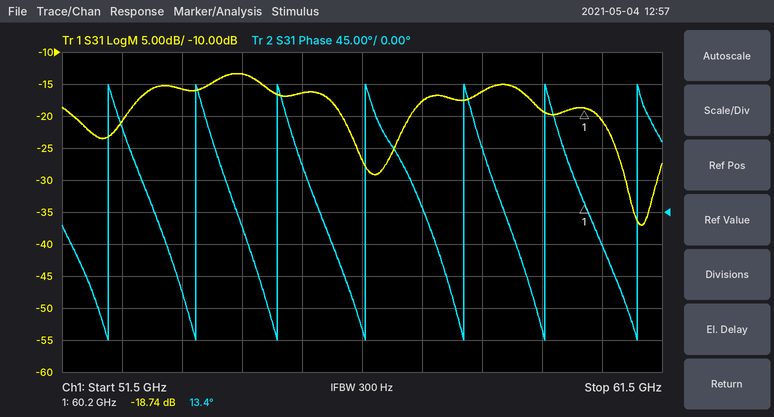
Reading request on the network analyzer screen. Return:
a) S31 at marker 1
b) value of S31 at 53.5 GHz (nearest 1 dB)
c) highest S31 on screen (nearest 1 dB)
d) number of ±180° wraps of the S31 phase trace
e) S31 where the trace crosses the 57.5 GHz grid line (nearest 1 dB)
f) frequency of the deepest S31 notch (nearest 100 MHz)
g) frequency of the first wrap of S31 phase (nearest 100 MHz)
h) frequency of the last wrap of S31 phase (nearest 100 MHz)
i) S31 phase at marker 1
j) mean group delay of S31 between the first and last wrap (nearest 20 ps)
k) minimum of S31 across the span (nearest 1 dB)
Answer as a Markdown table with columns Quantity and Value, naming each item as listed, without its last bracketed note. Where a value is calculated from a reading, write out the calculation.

| Quantity | Value |
|---|---|
| S31 at marker 1 | -18.74 dB |
| value of S31 at 53.5 GHz | -16 dB |
| highest S31 on screen | -13 dB |
| number of ±180° wraps of the S31 phase trace | 7 |
| S31 where the trace crosses the 57.5 GHz grid line | -18 dB |
| frequency of the deepest S31 notch | 61.2 GHz |
| frequency of the first wrap of S31 phase | 52.3 GHz |
| frequency of the last wrap of S31 phase | 61.1 GHz |
| S31 phase at marker 1 | 13.4° |
| mean group delay of S31 between the first and last wrap | 6 cycles / (61.1 GHz − 52.3 GHz) ≈ 682 ps, so 680 ps to the nearest 20 ps |
| minimum of S31 across the span | -37 dB |
